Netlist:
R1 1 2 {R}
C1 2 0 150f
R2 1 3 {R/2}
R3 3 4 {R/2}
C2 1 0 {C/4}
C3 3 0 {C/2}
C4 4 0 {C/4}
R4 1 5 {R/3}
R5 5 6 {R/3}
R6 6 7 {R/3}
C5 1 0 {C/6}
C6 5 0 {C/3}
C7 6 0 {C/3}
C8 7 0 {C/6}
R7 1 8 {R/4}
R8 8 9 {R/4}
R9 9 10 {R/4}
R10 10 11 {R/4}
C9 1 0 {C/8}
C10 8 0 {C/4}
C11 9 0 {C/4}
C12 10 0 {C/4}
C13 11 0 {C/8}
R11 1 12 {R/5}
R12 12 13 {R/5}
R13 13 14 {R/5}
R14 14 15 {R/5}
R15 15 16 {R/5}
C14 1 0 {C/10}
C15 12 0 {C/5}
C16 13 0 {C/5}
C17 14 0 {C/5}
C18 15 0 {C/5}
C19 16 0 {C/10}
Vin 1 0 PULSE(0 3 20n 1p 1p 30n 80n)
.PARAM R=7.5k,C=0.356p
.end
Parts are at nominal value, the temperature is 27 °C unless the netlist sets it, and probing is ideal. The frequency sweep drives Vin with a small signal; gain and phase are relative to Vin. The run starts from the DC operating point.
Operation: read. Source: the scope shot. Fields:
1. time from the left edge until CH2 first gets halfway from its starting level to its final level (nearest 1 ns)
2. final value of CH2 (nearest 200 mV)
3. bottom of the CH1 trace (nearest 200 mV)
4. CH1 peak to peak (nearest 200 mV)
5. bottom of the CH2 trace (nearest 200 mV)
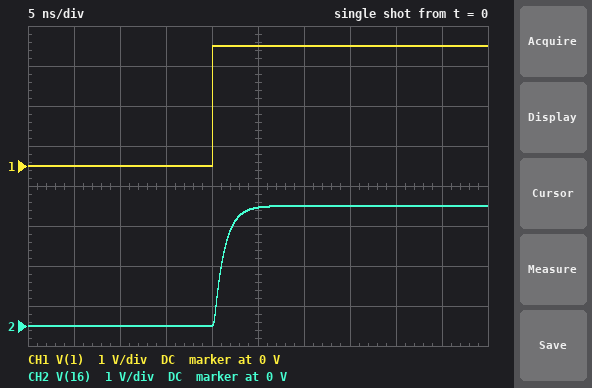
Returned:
21 ns
3.0 V
0 V
3.0 V
0 V
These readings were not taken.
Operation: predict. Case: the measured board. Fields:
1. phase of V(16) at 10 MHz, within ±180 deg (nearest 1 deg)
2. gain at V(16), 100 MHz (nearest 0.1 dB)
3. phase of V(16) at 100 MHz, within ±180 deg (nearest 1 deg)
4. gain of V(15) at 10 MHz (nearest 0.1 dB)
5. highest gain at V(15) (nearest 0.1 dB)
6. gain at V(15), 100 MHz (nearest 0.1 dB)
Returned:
-5 deg
-1.7 dB
-43 deg
0 dB
0 dB
-1.7 dB
